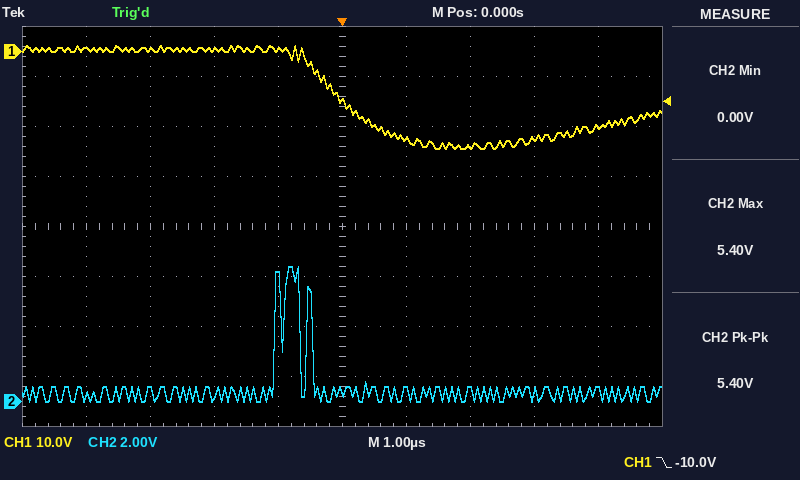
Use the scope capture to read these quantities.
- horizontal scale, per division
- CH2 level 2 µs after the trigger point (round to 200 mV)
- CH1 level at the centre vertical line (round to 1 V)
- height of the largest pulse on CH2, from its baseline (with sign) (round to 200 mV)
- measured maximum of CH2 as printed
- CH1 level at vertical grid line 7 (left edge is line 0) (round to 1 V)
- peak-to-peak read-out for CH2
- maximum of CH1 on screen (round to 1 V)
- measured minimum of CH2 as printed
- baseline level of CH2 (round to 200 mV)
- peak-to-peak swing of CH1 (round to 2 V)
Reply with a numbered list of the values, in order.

1. 1 µs
2. 400 mV
3. -10 V
4. +5.0 V
5. 5.40 V
6. -19 V
7. 5.40 V
8. 1 V
9. 0.00 V
10. 400 mV
11. 20 V
